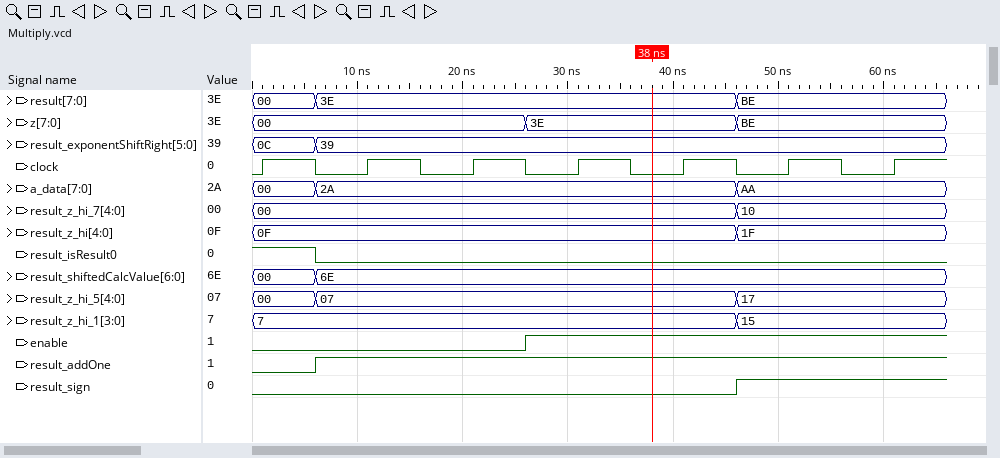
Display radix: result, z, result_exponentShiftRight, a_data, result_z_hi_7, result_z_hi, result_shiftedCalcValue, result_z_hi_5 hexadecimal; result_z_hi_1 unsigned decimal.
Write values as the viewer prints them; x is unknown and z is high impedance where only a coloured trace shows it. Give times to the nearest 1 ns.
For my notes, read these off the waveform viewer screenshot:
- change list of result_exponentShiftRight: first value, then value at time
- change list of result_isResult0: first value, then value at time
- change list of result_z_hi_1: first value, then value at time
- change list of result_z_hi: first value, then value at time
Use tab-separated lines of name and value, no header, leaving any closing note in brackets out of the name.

change list of result_exponentShiftRight: first value, then value at time	0C, 39 at 6 ns
change list of result_isResult0: first value, then value at time	1, 0 at 6 ns
change list of result_z_hi_1: first value, then value at time	7, 15 at 46 ns
change list of result_z_hi: first value, then value at time	0F, 1F at 46 ns
